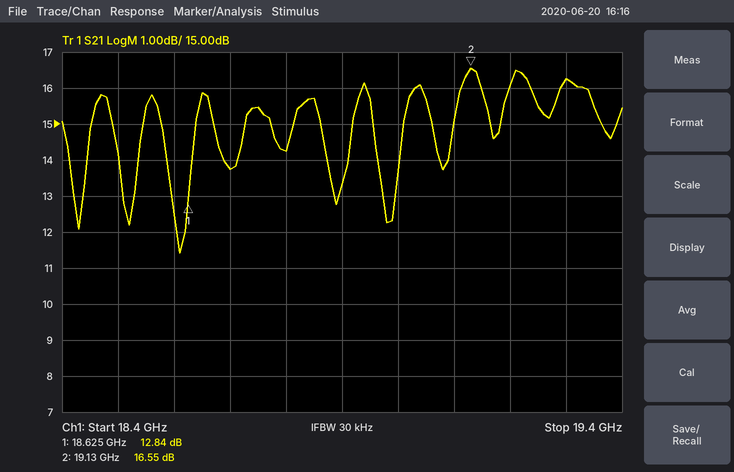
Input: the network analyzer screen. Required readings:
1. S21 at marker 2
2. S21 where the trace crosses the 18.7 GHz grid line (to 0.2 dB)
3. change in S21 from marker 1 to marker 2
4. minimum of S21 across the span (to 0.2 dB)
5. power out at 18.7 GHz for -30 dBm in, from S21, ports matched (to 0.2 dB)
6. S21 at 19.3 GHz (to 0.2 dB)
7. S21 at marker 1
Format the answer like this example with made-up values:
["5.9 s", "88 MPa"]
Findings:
["16.55 dB", "13.8 dB", "3.71 dB", "11.4 dB", "-16.2 dBm", "16.2 dB", "12.84 dB"]
